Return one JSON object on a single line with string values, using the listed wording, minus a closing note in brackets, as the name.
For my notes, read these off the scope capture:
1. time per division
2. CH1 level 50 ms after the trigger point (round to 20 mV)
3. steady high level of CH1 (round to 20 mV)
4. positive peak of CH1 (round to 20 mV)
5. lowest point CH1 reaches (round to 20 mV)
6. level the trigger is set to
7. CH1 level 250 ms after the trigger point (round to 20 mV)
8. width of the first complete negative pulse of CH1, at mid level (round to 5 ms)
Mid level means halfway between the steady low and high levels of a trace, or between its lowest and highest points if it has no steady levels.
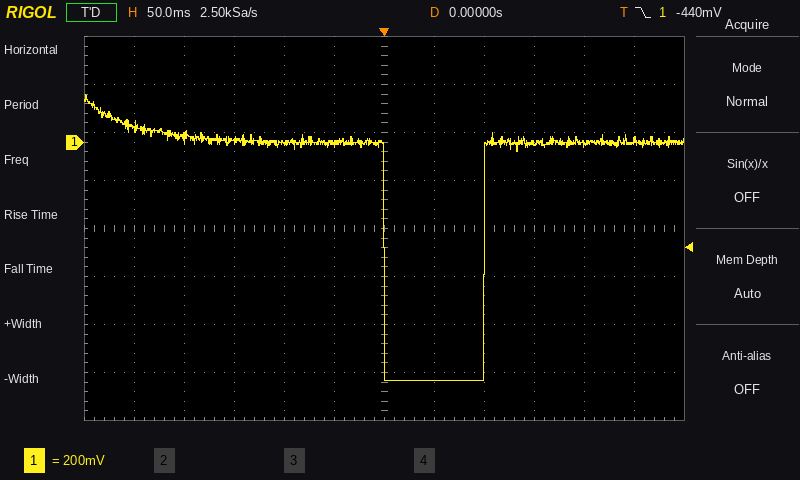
{"time per division": "50 ms", "CH1 level 50 ms after the trigger point": "-1.00 V", "steady high level of CH1": "0 mV", "positive peak of CH1": "200 mV", "lowest point CH1 reaches": "-1.00 V", "level the trigger is set to": "-440 mV", "CH1 level 250 ms after the trigger point": "0 mV", "width of the first complete negative pulse of CH1, at mid level": "100 ms"}
